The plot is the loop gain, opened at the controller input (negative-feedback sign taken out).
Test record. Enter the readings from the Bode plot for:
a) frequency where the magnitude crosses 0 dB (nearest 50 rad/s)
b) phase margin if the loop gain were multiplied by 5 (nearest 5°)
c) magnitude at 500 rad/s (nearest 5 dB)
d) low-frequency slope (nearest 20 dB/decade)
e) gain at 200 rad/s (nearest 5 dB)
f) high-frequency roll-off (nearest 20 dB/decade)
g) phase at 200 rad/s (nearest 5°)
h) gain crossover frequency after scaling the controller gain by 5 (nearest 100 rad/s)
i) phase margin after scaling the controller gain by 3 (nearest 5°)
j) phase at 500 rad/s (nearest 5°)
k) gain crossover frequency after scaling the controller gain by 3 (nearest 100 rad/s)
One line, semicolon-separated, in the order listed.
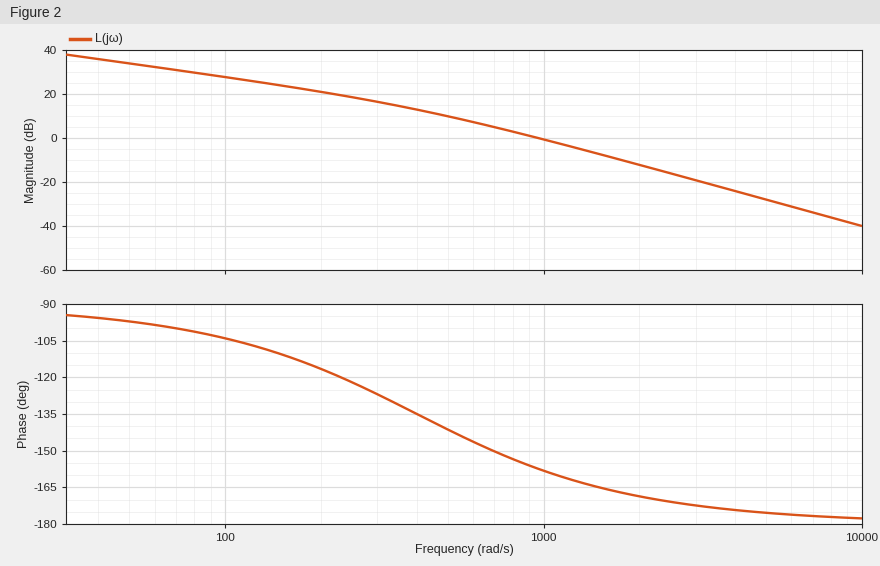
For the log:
950 rad/s; 10°; 10 dB; -20 dB/decade; 20 dB; -40 dB/decade; -115°; 2200 rad/s; 15°; -140°; 1700 rad/s
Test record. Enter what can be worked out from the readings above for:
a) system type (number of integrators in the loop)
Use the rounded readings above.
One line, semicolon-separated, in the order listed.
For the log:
1
